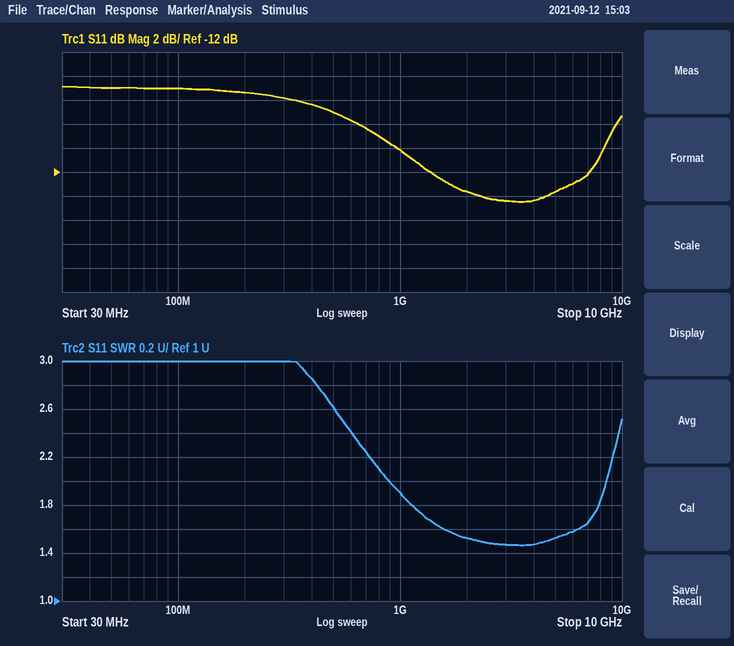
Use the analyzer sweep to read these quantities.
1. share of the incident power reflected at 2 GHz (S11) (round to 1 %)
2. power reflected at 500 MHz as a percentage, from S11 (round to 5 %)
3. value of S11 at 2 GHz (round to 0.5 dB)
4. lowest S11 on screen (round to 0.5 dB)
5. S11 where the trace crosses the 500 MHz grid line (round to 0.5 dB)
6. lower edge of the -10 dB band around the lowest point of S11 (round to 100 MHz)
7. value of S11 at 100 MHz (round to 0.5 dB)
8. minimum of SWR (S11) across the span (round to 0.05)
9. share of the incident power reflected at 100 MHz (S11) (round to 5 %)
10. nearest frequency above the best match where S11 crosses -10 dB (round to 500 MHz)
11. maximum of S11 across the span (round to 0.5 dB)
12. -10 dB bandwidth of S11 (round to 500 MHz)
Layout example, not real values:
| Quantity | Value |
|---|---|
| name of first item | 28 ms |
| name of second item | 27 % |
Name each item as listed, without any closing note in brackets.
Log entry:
| Quantity | Value |
|---|---|
| share of the incident power reflected at 2 GHz (S11) | 4 % |
| power reflected at 500 MHz as a percentage, from S11 | 20 % |
| value of S11 at 2 GHz | -13.5 dB |
| lowest S11 on screen | -14.5 dB |
| S11 where the trace crosses the 500 MHz grid line | -7.0 dB |
| lower edge of the -10 dB band around the lowest point of S11 | 1.0 GHz |
| value of S11 at 100 MHz | -5.0 dB |
| minimum of SWR (S11) across the span | 1.45 |
| share of the incident power reflected at 100 MHz (S11) | 30 % |
| nearest frequency above the best match where S11 crosses -10 dB | 8.5 GHz |
| maximum of S11 across the span | -5.0 dB |
| -10 dB bandwidth of S11 | 7.5 GHz |
